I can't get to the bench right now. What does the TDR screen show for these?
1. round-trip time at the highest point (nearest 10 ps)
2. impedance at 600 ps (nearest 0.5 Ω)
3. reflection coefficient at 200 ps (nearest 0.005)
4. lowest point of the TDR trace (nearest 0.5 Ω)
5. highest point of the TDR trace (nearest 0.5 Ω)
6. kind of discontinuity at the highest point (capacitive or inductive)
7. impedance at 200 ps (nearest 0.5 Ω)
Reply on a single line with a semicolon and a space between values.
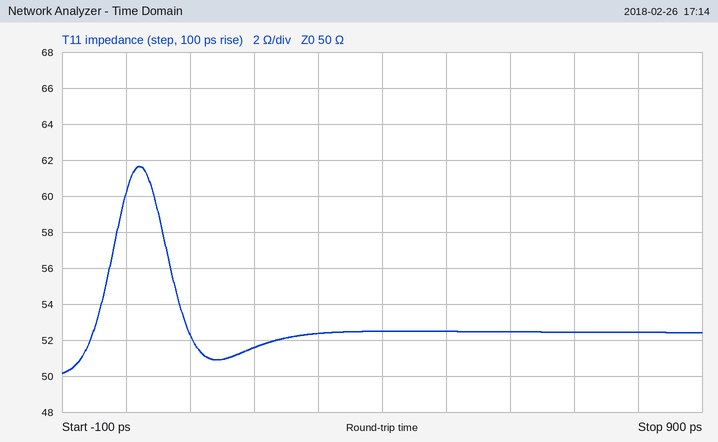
20 ps; 52.5 Ω; +0.015; 50.0 Ω; 61.5 Ω; inductive; 51.5 Ω
